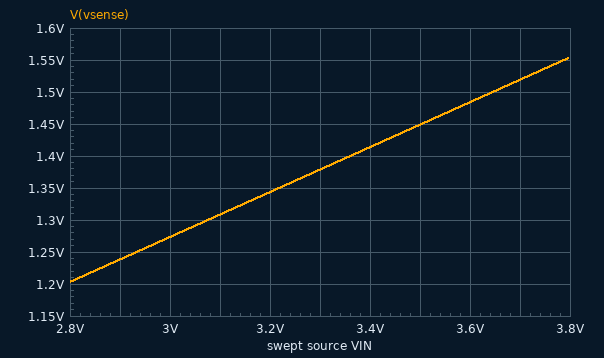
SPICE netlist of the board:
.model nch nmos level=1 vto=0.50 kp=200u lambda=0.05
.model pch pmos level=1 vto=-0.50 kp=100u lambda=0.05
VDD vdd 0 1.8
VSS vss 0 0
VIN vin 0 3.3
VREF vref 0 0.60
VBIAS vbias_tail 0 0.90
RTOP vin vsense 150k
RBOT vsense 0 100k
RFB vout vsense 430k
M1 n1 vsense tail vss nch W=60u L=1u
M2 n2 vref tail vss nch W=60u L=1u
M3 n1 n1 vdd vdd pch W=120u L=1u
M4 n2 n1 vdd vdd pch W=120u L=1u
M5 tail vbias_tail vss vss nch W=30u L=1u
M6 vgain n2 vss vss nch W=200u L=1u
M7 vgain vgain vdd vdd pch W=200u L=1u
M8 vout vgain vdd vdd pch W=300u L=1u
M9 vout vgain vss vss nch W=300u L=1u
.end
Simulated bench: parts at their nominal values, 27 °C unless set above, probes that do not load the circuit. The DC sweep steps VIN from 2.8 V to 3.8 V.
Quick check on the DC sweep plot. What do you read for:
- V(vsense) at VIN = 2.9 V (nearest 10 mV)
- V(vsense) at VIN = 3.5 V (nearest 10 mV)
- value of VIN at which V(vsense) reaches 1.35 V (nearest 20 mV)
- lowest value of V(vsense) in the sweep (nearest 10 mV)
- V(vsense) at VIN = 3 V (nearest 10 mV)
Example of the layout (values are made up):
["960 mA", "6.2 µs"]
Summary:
["1.24 V", "1.45 V", "3.22 V", "1.20 V", "1.27 V"]
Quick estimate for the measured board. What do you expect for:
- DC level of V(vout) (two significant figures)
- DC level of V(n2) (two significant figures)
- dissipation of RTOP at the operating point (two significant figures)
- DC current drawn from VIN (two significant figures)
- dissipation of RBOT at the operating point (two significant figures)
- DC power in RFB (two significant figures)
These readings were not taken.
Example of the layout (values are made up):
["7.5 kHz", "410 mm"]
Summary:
["1.8 V", "1.8 V", "25 µW", "13 µA", "19 µW", "410 nW"]
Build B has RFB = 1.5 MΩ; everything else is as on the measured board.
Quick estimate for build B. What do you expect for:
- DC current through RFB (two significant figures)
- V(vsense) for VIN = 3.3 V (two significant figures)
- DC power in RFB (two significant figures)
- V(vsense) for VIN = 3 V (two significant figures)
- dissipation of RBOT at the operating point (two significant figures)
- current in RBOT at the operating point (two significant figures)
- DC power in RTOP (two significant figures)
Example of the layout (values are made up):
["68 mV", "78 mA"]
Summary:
["310 nA", "1.3 V", "140 nW", "1.2 V", "18 µW", "13 µA", "26 µW"]
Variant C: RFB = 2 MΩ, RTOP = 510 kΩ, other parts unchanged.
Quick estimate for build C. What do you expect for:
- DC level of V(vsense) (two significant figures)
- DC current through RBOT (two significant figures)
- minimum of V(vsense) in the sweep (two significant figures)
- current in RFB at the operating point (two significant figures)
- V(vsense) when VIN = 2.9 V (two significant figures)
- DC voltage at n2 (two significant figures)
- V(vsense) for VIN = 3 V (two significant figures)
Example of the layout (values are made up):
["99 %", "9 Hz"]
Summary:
["520 mV", "5.2 µA", "440 mV", "260 nA", "460 mV", "3.5 mV", "470 mV"]
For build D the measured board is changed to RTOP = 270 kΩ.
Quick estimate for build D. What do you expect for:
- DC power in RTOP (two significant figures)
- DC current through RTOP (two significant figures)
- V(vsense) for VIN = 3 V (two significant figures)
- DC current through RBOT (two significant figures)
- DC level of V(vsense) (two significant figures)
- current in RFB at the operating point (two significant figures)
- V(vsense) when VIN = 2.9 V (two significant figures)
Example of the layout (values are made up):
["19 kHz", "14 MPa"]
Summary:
["19 µW", "8.4 µA", "950 mV", "10 µA", "1.0 V", "1.8 µA", "930 mV"]
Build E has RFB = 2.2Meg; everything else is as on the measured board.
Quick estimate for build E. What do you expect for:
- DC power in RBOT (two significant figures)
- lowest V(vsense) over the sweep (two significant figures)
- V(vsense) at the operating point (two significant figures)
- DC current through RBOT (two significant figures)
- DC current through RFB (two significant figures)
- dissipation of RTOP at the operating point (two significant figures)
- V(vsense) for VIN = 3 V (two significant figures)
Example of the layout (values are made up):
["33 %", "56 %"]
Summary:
["18 µW", "1.1 V", "1.3 V", "13 µA", "210 nA", "26 µW", "1.2 V"]
